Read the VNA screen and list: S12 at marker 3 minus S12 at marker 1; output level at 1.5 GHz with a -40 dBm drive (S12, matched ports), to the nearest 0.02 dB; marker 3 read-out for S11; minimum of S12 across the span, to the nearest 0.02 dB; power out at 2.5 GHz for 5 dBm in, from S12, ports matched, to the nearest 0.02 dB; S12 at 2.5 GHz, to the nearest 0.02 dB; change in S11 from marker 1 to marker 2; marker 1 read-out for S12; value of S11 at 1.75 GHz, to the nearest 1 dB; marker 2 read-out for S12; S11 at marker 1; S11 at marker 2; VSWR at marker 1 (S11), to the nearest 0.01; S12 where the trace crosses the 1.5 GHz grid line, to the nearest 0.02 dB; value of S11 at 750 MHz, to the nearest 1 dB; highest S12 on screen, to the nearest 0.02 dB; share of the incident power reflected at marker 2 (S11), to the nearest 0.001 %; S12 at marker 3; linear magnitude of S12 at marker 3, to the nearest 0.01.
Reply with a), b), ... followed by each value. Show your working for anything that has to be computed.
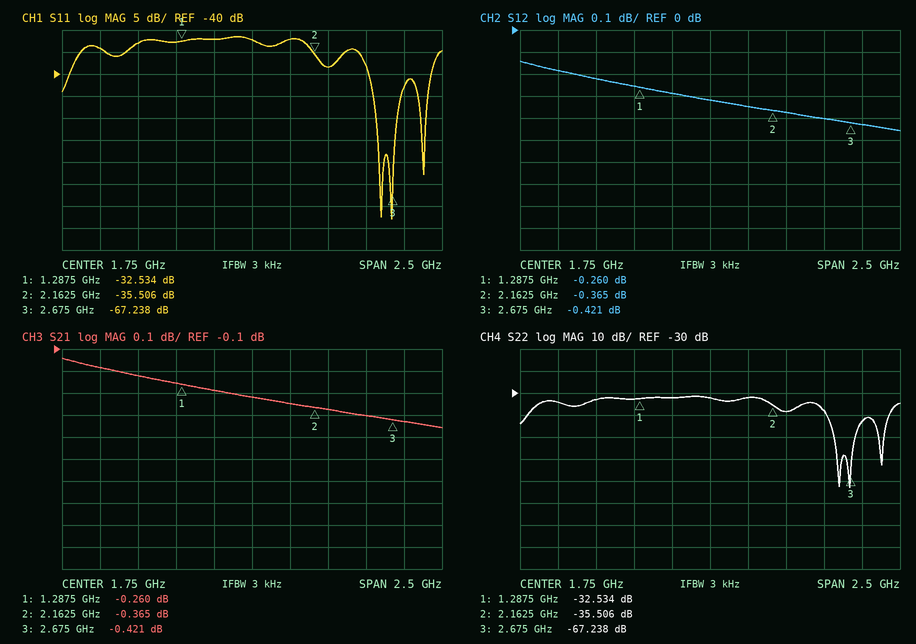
a) -0.421 − (-0.26) = -0.161 dB
b) -40 dBm + (-0.28 dB) = -40.28 dBm
c) -67.238 dB
d) -0.46 dB
e) 5 dBm + (-0.40 dB) = 4.60 dBm
f) -0.40 dB
g) -35.506 − (-32.534) = -2.972 dB
h) -0.260 dB
i) -32 dB
j) -0.365 dB
k) -32.534 dB
l) -35.506 dB
m) (1 + 0.0236)/(1 − 0.0236) ≈ 1.05
n) -0.28 dB
o) -34 dB
p) -0.14 dB
q) 10^(-35.506/10) ≈ 0.028 %
r) -0.421 dB
s) 10^(-0.421/20) ≈ 0.95
